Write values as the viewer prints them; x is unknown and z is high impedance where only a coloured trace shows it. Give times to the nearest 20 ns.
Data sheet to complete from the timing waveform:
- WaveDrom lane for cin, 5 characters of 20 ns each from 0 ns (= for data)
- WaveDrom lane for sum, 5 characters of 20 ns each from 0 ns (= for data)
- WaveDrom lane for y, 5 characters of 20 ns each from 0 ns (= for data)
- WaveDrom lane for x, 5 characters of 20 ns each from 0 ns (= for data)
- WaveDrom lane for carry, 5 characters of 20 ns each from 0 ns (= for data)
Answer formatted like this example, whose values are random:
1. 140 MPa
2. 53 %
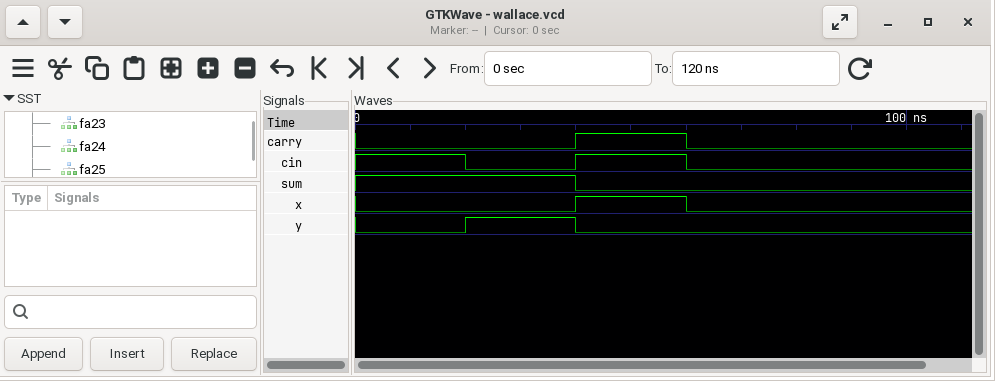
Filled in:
1. {name: 'cin', wave: '1010.'}
2. {name: 'sum', wave: '1.0..'}
3. {name: 'y', wave: '010..'}
4. {name: 'x', wave: '0.10.'}
5. {name: 'carry', wave: '0.10.'}
